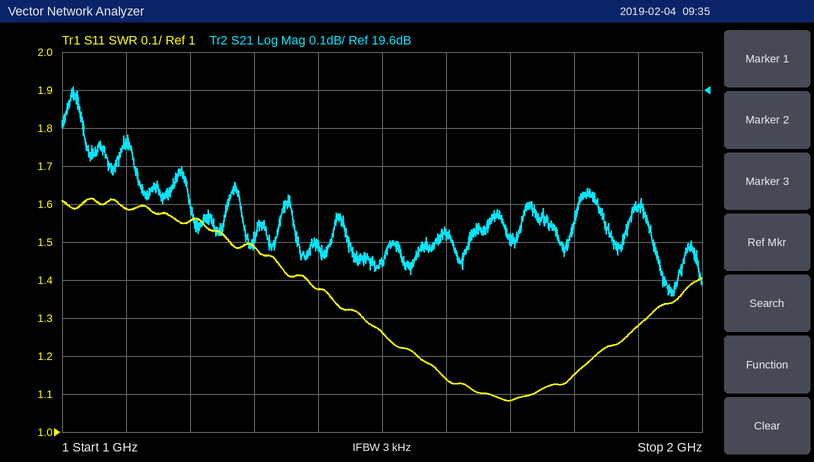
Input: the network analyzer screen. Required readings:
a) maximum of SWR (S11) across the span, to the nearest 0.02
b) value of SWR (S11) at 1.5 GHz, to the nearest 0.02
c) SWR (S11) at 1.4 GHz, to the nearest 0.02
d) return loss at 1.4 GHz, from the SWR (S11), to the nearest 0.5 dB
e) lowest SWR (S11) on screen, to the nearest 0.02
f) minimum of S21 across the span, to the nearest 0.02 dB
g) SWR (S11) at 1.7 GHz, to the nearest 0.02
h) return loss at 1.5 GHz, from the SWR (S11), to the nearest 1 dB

1.62
1.26
1.38
16.0 dB
1.08
19.06 dB
1.08
19 dB
